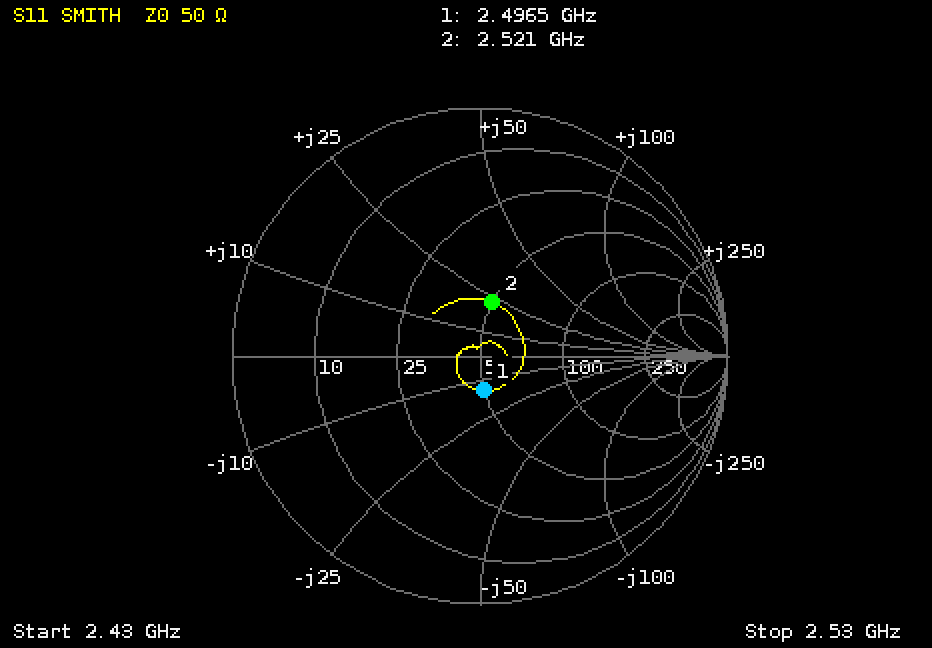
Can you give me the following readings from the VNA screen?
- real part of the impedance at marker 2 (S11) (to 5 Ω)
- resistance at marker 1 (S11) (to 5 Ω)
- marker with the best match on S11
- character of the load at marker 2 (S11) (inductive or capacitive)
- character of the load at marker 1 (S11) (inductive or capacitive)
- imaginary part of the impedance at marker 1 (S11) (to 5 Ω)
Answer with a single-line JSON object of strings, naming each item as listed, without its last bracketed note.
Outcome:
{"real part of the impedance at marker 2 (S11)": "50 Ω", "resistance at marker 1 (S11)": "50 Ω", "marker with the best match on S11": "marker 1", "character of the load at marker 2 (S11)": "inductive", "character of the load at marker 1 (S11)": "capacitive", "imaginary part of the impedance at marker 1 (S11)": "-15 Ω"}
